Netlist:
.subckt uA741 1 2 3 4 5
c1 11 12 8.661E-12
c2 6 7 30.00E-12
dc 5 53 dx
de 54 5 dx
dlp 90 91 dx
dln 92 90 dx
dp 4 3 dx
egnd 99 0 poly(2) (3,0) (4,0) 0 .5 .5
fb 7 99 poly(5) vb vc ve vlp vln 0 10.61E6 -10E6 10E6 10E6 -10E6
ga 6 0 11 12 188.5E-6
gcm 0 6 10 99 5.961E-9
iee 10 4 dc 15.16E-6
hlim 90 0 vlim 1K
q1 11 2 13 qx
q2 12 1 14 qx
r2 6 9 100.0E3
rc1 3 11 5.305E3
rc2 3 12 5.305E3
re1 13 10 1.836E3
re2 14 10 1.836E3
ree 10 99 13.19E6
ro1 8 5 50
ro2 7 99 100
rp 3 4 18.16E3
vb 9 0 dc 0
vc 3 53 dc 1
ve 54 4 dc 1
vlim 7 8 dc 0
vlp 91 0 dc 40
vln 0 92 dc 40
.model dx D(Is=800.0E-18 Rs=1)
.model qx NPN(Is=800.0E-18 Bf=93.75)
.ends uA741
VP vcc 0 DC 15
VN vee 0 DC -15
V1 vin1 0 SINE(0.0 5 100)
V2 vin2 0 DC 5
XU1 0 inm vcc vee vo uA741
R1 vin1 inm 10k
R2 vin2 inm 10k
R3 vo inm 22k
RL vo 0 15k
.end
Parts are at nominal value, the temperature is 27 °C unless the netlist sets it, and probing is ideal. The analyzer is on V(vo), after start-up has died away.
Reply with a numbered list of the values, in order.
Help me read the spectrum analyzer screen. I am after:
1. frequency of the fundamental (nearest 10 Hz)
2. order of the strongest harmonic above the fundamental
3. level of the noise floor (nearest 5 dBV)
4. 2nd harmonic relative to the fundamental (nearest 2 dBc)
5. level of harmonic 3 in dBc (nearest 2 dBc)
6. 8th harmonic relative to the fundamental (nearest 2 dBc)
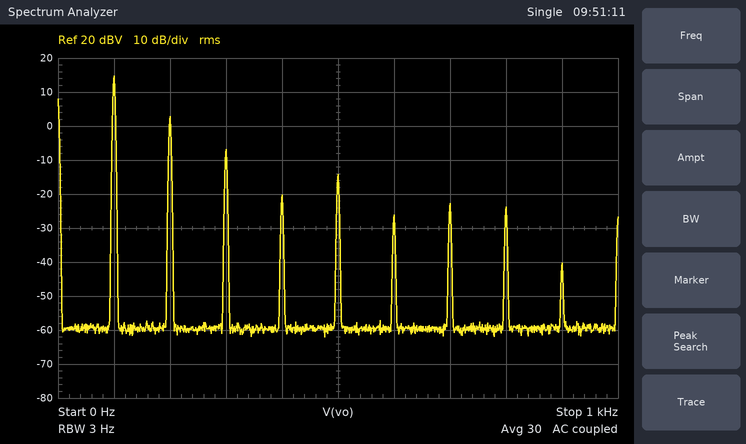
1. 100 Hz
2. 2
3. -60 dBV
4. -12 dBc
5. -22 dBc
6. -38 dBc
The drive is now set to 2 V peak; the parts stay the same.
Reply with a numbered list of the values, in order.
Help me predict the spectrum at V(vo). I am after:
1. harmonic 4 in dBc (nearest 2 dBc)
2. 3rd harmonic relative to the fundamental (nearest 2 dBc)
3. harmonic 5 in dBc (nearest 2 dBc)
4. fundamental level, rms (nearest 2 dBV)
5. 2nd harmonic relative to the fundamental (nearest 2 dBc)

1. -32 dBc
2. -30 dBc
3. -36 dBc
4. 10 dBV
5. -28 dBc
